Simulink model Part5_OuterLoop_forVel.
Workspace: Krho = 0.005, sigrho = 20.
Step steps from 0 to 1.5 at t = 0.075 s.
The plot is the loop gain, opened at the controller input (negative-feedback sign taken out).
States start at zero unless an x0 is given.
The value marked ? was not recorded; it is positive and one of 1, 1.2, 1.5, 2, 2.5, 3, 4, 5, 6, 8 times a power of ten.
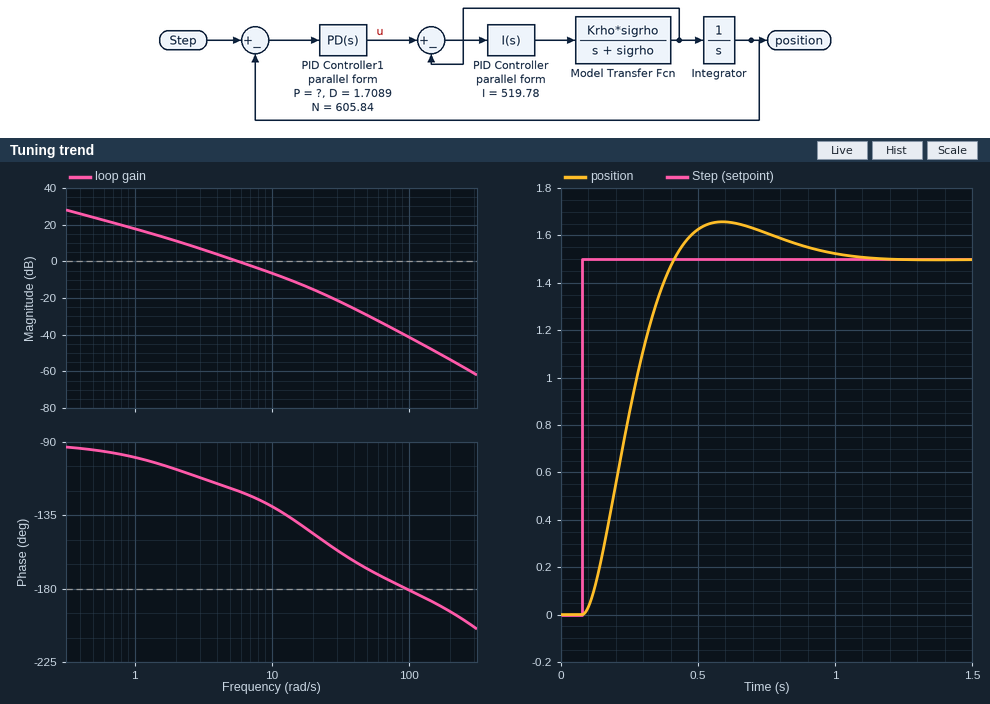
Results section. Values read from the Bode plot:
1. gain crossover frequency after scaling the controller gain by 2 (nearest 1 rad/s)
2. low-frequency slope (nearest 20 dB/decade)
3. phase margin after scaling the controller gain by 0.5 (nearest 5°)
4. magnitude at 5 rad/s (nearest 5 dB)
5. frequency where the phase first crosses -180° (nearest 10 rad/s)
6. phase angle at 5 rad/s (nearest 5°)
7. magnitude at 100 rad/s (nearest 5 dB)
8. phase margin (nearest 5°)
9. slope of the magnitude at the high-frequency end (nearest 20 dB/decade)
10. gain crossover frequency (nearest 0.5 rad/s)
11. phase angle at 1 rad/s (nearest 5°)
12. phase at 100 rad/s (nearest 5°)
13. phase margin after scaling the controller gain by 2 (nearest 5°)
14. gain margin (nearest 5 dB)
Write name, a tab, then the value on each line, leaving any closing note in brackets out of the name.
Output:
gain crossover frequency after scaling the controller gain by 2	10 rad/s
low-frequency slope	-20 dB/decade
phase margin after scaling the controller gain by 0.5	65°
magnitude at 5 rad/s	0 dB
frequency where the phase first crosses -180°	100 rad/s
phase angle at 5 rad/s	-120°
magnitude at 100 rad/s	-40 dB
phase margin	60°
slope of the magnitude at the high-frequency end	-40 dB/decade
gain crossover frequency	5.5 rad/s
phase angle at 1 rad/s	-100°
phase at 100 rad/s	-180°
phase margin after scaling the controller gain by 2	50°
gain margin	40 dB
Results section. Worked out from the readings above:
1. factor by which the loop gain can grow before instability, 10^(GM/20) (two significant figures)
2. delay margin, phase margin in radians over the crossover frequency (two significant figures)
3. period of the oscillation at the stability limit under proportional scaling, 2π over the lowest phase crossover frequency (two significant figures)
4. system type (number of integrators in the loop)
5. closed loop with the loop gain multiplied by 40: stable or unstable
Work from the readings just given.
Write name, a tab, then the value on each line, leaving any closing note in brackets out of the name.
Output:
factor by which the loop gain can grow before instability, 10^(GM/20)	100
delay margin, phase margin in radians over the crossover frequency	0.19 s
period of the oscillation at the stability limit under proportional scaling, 2π over the lowest phase crossover frequency	0.063 s
system type	1
closed loop with the loop gain multiplied by 40: stable or unstable	stable
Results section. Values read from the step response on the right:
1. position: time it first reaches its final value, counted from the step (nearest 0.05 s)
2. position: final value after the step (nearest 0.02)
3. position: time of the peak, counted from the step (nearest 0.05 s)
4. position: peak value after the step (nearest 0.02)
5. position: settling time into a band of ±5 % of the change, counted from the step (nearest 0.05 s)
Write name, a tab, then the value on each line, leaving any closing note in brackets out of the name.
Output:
position: time it first reaches its final value, counted from the step	0.35 s
position: final value after the step	1.50
position: time of the peak, counted from the step	0.50 s
position: peak value after the step	1.66
position: settling time into a band of ±5 % of the change, counted from the step	0.75 s
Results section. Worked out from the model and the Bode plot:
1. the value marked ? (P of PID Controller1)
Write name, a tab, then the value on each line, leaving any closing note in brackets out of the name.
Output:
the value marked ?	8
